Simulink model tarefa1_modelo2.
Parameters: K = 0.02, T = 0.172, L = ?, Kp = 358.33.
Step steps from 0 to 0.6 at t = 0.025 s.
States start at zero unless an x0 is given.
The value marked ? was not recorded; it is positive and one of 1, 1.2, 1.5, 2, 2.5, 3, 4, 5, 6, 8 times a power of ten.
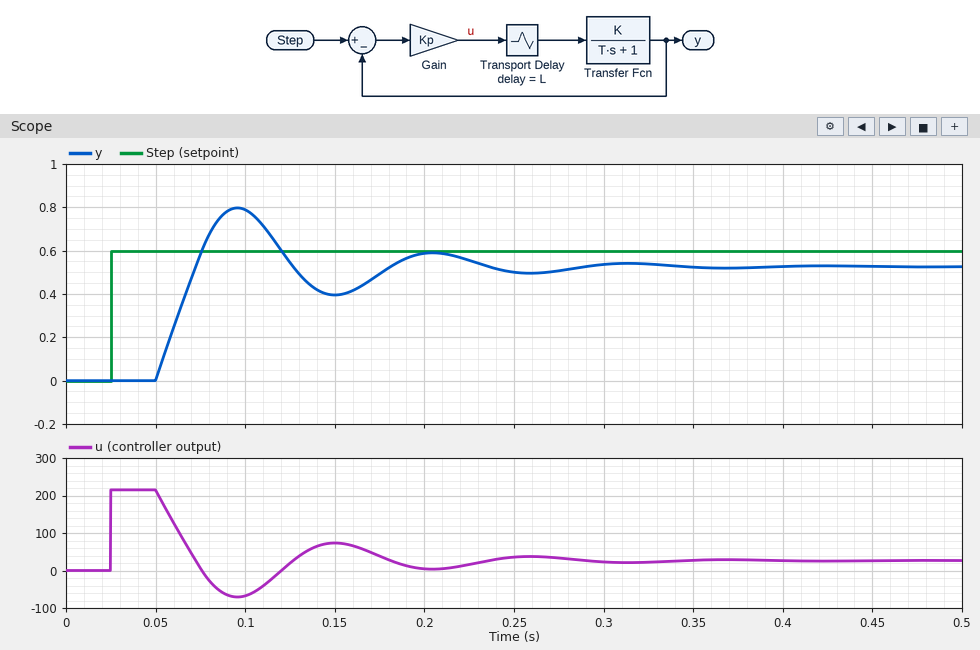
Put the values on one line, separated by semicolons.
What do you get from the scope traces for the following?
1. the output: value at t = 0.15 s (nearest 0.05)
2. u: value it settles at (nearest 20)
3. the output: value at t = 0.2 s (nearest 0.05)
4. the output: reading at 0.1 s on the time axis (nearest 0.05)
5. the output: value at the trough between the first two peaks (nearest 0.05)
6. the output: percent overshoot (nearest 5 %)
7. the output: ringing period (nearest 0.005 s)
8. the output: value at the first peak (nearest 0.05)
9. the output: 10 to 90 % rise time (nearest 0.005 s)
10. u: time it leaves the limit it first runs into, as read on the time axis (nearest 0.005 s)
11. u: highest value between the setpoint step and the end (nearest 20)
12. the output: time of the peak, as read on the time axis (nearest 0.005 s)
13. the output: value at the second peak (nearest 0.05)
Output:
0.40; 20; 0.60; 0.80; 0.40; 50 %; 0.110 s; 0.80; 0.020 s; 0.050 s; 220; 0.095 s; 0.60
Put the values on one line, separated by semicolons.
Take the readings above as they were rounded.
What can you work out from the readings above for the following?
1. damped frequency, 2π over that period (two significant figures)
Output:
57 rad/s
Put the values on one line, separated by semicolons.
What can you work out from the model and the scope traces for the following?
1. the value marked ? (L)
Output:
0.025
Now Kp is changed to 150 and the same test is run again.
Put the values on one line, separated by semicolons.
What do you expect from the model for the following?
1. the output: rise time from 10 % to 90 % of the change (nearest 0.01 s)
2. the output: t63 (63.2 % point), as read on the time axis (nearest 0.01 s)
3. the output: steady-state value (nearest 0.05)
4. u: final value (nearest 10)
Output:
0.05 s; 0.08 s; 0.45; 20
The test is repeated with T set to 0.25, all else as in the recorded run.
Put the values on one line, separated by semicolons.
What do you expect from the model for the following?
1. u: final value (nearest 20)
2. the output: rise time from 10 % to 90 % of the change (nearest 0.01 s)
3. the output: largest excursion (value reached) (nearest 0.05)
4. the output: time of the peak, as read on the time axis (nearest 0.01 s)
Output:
20; 0.03 s; 0.65; 0.11 s
